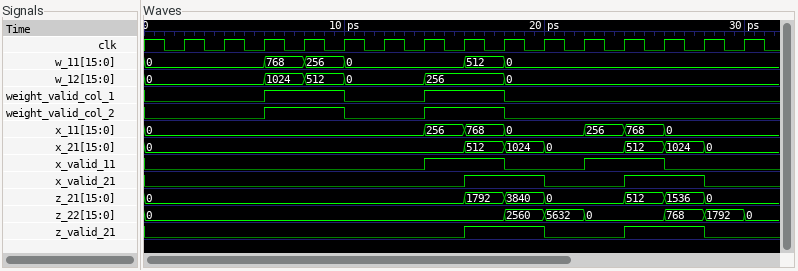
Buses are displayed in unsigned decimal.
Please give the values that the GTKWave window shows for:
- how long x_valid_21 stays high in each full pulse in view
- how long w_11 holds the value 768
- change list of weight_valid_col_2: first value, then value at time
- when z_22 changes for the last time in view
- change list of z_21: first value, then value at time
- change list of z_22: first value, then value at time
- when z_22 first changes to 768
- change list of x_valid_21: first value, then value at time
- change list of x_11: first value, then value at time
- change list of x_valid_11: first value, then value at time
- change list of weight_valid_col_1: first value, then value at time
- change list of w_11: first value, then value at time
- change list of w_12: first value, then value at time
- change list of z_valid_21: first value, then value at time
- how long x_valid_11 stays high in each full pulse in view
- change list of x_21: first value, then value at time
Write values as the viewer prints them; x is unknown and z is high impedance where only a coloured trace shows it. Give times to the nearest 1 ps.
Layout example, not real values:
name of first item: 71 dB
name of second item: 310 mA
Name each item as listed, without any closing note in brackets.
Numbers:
how long x_valid_21 stays high in each full pulse in view: 4 ps, 4 ps
how long w_11 holds the value 768: 2 ps
change list of weight_valid_col_2: first value, then value at time: 0, 1 at 6 ps, 0 at 10 ps, 1 at 14 ps, 0 at 18 ps
when z_22 changes for the last time in view: 30 ps
change list of z_21: first value, then value at time: 0, 1792 at 16 ps, 3840 at 18 ps, 0 at 20 ps, 512 at 24 ps, 1536 at 26 ps, 0 at 28 ps
change list of z_22: first value, then value at time: 0, 2560 at 18 ps, 5632 at 20 ps, 0 at 22 ps, 768 at 26 ps, 1792 at 28 ps, 0 at 30 ps
when z_22 first changes to 768: 26 ps
change list of x_valid_21: first value, then value at time: 0, 1 at 16 ps, 0 at 20 ps, 1 at 24 ps, 0 at 28 ps
change list of x_11: first value, then value at time: 0, 256 at 14 ps, 768 at 16 ps, 0 at 18 ps, 256 at 22 ps, 768 at 24 ps, 0 at 26 ps
change list of x_valid_11: first value, then value at time: 0, 1 at 14 ps, 0 at 18 ps, 1 at 22 ps, 0 at 26 ps
change list of weight_valid_col_1: first value, then value at time: 0, 1 at 6 ps, 0 at 10 ps, 1 at 14 ps, 0 at 18 ps
change list of w_11: first value, then value at time: 0, 768 at 6 ps, 256 at 8 ps, 0 at 10 ps, 512 at 16 ps, 0 at 18 ps
change list of w_12: first value, then value at time: 0, 1024 at 6 ps, 512 at 8 ps, 0 at 10 ps, 256 at 14 ps, 0 at 18 ps
change list of z_valid_21: first value, then value at time: 0, 1 at 16 ps, 0 at 20 ps, 1 at 24 ps, 0 at 28 ps
how long x_valid_11 stays high in each full pulse in view: 4 ps, 4 ps
change list of x_21: first value, then value at time: 0, 512 at 16 ps, 1024 at 18 ps, 0 at 20 ps, 512 at 24 ps, 1024 at 26 ps, 0 at 28 ps
